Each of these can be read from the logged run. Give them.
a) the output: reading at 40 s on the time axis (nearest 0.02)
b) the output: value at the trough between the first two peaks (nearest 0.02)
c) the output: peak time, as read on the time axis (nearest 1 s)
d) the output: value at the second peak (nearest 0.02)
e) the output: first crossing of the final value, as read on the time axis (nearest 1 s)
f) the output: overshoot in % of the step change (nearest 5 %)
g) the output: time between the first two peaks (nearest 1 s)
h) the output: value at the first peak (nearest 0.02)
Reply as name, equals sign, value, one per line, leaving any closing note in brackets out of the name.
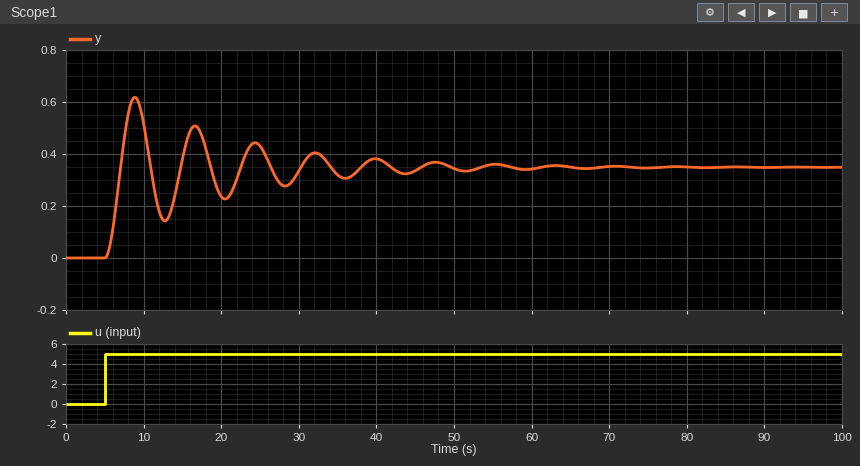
the output: reading at 40 s on the time axis = 0.38
the output: value at the trough between the first two peaks = 0.14
the output: peak time, as read on the time axis = 9 s
the output: value at the second peak = 0.50
the output: first crossing of the final value, as read on the time axis = 7 s
the output: overshoot in % of the step change = 75 %
the output: time between the first two peaks = 8 s
the output: value at the first peak = 0.62
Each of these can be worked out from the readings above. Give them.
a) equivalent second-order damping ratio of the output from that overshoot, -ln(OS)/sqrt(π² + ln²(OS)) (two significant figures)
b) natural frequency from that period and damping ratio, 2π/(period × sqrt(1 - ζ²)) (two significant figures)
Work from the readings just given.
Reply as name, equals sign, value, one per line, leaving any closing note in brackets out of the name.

equivalent second-order damping ratio of the output from that overshoot, -ln(OS)/sqrt(π² + ln²(OS)) = 0.091
natural frequency from that period and damping ratio, 2π/(period × sqrt(1 - ζ²)) = 0.79 rad/s
